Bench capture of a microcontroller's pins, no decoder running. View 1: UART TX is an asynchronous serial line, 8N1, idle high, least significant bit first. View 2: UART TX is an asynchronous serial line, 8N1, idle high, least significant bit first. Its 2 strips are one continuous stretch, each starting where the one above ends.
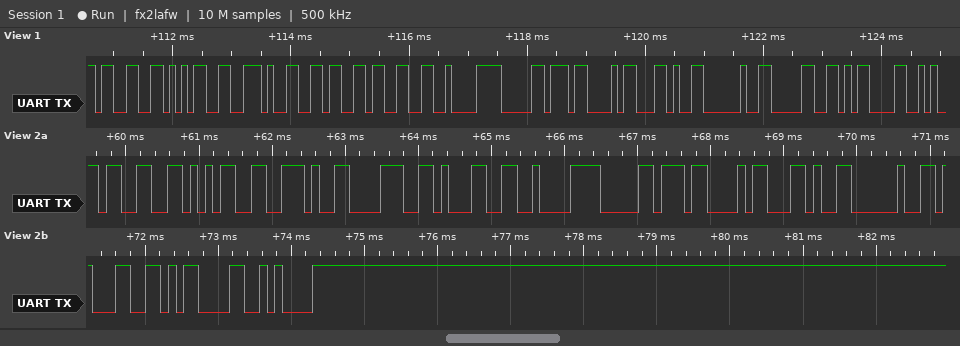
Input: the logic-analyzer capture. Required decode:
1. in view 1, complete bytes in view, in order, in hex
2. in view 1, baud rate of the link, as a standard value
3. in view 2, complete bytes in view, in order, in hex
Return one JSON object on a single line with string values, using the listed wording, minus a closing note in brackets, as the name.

{"in view 1, complete bytes in view, in order, in hex": "33 35 2E 36 33 C2 B0 43 2C 20 30 0D", "in view 1, baud rate of the link, as a standard value": "9600 baud", "in view 2, complete bytes in view, in order, in hex": "33 35 2E 38 31 C2 B0 43 2C 20 31 0D 0A"}
